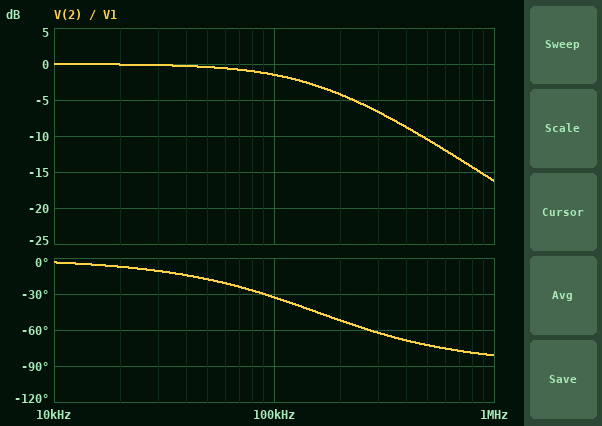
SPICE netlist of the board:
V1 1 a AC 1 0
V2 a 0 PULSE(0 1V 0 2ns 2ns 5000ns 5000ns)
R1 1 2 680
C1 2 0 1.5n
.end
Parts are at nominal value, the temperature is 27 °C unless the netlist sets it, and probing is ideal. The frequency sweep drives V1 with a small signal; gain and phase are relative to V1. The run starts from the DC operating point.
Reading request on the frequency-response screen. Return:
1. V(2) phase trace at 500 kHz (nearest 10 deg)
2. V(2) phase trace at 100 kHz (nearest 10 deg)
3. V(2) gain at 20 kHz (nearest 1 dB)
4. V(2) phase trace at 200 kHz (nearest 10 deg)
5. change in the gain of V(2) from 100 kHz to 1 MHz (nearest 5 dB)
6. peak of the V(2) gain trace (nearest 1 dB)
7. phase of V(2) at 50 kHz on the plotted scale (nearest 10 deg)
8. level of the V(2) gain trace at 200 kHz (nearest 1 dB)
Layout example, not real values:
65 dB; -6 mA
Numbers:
-70 deg; -30 deg; 0 dB; -50 deg; -15 dB; 0 dB; -20 deg; -4 dB
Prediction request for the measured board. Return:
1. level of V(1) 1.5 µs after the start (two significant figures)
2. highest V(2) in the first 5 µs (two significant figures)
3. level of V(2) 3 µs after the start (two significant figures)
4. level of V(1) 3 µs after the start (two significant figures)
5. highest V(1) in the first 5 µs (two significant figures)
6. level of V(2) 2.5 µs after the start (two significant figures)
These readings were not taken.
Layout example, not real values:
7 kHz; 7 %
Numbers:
1.0 V; 990 mV; 950 mV; 1.0 V; 1.0 V; 910 mV
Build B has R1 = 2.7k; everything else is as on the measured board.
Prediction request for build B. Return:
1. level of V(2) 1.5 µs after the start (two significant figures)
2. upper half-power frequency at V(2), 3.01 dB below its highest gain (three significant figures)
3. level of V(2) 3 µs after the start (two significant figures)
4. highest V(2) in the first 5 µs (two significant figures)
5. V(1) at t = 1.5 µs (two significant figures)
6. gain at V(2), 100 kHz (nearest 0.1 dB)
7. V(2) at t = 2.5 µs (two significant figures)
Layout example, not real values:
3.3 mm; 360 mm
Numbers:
310 mV; 39.3 kHz; 520 mV; 710 mV; 1.0 V; -8.7 dB; 460 mV
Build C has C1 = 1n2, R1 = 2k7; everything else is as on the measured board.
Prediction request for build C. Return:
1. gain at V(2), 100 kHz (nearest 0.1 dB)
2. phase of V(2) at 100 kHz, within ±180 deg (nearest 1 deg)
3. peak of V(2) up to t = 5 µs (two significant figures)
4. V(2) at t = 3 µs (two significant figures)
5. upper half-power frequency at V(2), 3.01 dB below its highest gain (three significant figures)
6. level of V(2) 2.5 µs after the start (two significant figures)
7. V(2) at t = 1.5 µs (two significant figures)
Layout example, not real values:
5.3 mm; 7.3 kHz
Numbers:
-7.1 dB; -64 deg; 790 mV; 600 mV; 49.1 kHz; 540 mV; 370 mV
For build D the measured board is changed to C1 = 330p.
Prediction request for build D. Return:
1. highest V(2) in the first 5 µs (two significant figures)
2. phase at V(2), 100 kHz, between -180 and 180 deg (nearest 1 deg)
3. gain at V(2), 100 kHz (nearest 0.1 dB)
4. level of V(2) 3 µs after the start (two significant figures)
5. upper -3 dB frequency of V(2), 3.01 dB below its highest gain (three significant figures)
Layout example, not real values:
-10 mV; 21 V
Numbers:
1.0 V; -8 deg; -0.1 dB; 1.0 V; 709 kHz
